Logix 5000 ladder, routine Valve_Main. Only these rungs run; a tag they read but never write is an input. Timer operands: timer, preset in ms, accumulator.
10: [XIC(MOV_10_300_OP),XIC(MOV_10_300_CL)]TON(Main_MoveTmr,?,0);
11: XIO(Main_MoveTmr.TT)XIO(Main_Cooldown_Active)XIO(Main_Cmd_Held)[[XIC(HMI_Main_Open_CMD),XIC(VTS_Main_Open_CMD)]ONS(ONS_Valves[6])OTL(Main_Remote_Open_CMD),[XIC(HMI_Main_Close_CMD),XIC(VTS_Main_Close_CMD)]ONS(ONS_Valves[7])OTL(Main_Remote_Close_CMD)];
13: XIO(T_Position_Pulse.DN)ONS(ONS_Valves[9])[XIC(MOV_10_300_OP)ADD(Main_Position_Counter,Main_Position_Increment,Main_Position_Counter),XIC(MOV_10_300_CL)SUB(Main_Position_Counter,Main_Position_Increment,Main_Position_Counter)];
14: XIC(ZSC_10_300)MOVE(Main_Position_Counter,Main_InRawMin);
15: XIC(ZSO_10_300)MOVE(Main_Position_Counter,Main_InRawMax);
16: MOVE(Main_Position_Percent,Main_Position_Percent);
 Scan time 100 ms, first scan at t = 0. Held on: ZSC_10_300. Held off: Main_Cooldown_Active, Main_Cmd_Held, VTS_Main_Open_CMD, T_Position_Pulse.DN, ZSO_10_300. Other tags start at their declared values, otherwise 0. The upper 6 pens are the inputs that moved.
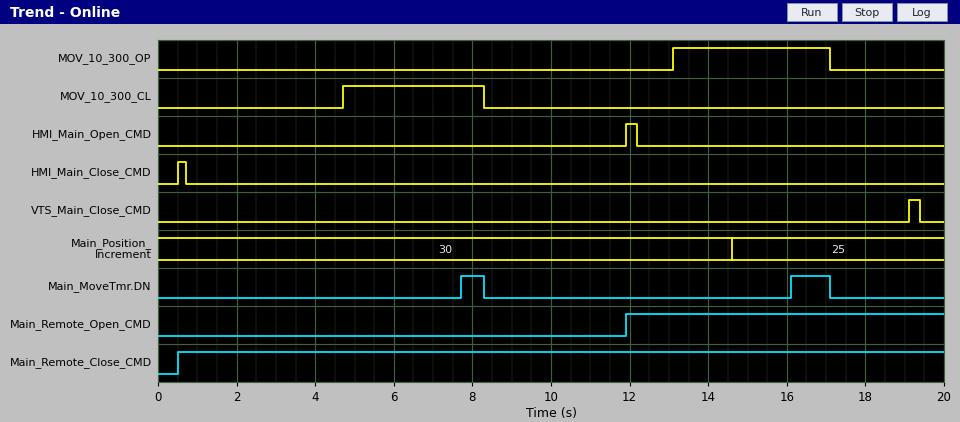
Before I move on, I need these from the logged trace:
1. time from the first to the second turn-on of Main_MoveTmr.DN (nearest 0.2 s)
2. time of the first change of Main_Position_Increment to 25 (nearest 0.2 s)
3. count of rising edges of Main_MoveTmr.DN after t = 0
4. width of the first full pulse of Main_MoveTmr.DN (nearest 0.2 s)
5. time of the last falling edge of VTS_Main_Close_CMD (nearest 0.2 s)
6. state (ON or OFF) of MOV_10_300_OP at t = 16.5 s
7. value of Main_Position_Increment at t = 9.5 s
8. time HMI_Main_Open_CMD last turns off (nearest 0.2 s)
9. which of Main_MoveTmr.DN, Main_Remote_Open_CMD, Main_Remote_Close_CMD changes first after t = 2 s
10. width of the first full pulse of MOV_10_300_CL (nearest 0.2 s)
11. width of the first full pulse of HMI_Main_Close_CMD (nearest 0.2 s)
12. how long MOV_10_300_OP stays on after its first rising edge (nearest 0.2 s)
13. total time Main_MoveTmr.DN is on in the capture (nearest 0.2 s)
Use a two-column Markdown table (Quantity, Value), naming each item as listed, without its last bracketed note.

| Quantity | Value |
|---|---|
| time from the first to the second turn-on of Main_MoveTmr.DN | 8.4 s |
| time of the first change of Main_Position_Increment to 25 | 14.6 s |
| count of rising edges of Main_MoveTmr.DN after t = 0 | 2 |
| width of the first full pulse of Main_MoveTmr.DN | 0.6 s |
| time of the last falling edge of VTS_Main_Close_CMD | 19.4 s |
| state (ON or OFF) of MOV_10_300_OP at t = 16.5 s | ON |
| value of Main_Position_Increment at t = 9.5 s | 30 |
| time HMI_Main_Open_CMD last turns off | 12.2 s |
| which of Main_MoveTmr.DN, Main_Remote_Open_CMD, Main_Remote_Close_CMD changes first after t = 2 s | Main_MoveTmr.DN |
| width of the first full pulse of MOV_10_300_CL | 3.6 s |
| width of the first full pulse of HMI_Main_Close_CMD | 0.2 s |
| how long MOV_10_300_OP stays on after its first rising edge | 4.0 s |
| total time Main_MoveTmr.DN is on in the capture | 1.6 s |
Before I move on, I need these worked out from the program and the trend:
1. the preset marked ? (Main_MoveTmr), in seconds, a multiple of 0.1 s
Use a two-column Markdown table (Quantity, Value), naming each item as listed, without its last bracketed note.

| Quantity | Value |
|---|---|
| the preset marked ? (Main_MoveTmr), in seconds, a multiple of 0.1 s | 3.0 s |
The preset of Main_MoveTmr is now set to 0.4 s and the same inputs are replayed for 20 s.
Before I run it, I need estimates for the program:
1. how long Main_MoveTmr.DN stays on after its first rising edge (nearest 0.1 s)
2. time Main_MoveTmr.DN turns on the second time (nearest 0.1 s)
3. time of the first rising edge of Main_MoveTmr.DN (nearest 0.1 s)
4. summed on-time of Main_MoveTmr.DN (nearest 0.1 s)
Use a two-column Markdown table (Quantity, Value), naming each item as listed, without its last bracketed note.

| Quantity | Value |
|---|---|
| how long Main_MoveTmr.DN stays on after its first rising edge | 3.2 s |
| time Main_MoveTmr.DN turns on the second time | 13.5 s |
| time of the first rising edge of Main_MoveTmr.DN | 5.1 s |
| summed on-time of Main_MoveTmr.DN | 6.8 s |
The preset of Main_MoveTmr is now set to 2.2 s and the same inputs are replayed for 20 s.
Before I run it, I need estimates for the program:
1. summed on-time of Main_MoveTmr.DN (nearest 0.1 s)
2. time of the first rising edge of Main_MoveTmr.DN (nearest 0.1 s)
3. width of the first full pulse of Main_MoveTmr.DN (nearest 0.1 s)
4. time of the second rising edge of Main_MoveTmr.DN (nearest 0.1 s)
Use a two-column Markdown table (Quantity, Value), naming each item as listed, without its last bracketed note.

| Quantity | Value |
|---|---|
| summed on-time of Main_MoveTmr.DN | 3.2 s |
| time of the first rising edge of Main_MoveTmr.DN | 6.9 s |
| width of the first full pulse of Main_MoveTmr.DN | 1.4 s |
| time of the second rising edge of Main_MoveTmr.DN | 15.3 s |
